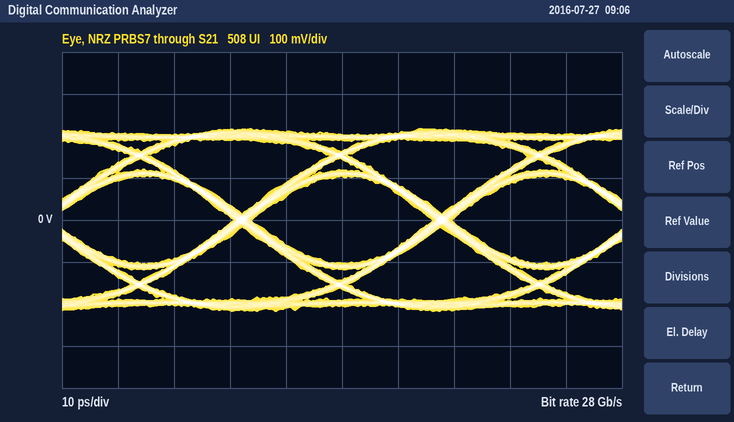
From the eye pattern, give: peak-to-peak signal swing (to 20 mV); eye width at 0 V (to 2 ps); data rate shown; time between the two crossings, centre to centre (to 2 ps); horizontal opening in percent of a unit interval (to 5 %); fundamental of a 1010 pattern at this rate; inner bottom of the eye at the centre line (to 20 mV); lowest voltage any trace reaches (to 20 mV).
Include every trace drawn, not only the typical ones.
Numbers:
440 mV
32 ps
28 Gb/s
36 ps
90 %
14 GHz
-100 mV
-220 mV
